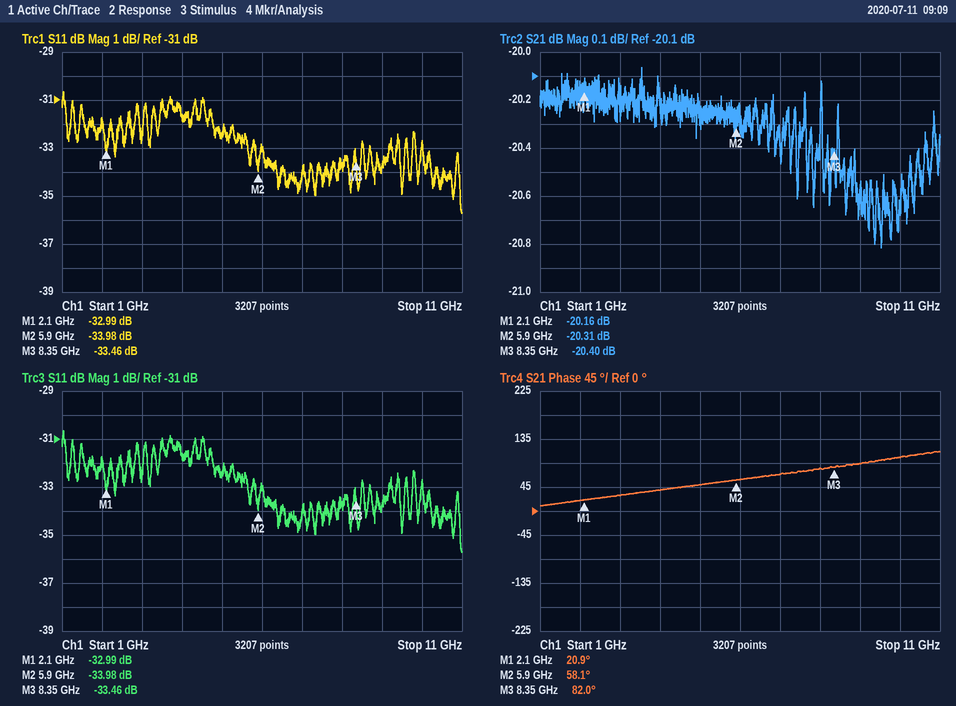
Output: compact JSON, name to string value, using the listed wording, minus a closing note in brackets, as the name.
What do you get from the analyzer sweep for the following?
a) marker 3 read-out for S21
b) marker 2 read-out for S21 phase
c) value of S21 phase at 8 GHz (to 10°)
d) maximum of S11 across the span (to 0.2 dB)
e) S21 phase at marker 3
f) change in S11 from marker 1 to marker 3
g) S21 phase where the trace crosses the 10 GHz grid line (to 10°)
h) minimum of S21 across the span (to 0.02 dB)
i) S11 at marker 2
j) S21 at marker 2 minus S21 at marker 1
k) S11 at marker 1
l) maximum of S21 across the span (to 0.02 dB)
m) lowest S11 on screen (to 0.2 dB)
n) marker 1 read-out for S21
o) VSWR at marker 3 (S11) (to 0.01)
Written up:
{"marker 3 read-out for S21": "-20.40 dB", "marker 2 read-out for S21 phase": "58.1°", "value of S21 phase at 8 GHz": "80°", "maximum of S11 across the span": "-30.6 dB", "S21 phase at marker 3": "82.0°", "change in S11 from marker 1 to marker 3": "-0.47 dB", "S21 phase where the trace crosses the 10 GHz grid line": "100°", "minimum of S21 across the span": "-20.82 dB", "S11 at marker 2": "-33.98 dB", "S21 at marker 2 minus S21 at marker 1": "-0.15 dB", "S11 at marker 1": "-32.99 dB", "maximum of S21 across the span": "-20.06 dB", "lowest S11 on screen": "-35.8 dB", "marker 1 read-out for S21": "-20.16 dB", "VSWR at marker 3 (S11)": "1.04"}
